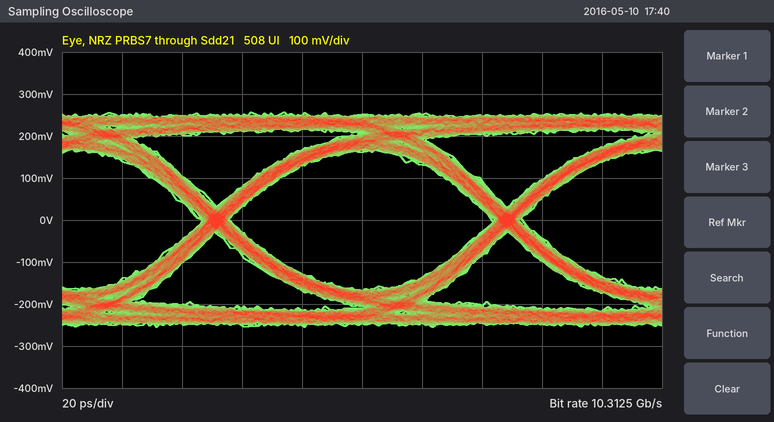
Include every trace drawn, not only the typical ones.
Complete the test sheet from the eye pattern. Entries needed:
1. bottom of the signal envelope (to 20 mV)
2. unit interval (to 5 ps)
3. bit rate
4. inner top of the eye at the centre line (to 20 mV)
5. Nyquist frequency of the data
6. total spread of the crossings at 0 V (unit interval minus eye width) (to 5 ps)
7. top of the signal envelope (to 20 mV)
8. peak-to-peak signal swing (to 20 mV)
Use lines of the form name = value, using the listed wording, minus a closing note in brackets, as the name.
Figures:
bottom of the signal envelope = -260 mV
unit interval = 95 ps
bit rate = 10.3125 Gb/s
inner top of the eye at the centre line = 160 mV
Nyquist frequency of the data = 5.15625 GHz
total spread of the crossings at 0 V (unit interval minus eye width) = 10 ps
top of the signal envelope = 260 mV
peak-to-peak signal swing = 520 mV
